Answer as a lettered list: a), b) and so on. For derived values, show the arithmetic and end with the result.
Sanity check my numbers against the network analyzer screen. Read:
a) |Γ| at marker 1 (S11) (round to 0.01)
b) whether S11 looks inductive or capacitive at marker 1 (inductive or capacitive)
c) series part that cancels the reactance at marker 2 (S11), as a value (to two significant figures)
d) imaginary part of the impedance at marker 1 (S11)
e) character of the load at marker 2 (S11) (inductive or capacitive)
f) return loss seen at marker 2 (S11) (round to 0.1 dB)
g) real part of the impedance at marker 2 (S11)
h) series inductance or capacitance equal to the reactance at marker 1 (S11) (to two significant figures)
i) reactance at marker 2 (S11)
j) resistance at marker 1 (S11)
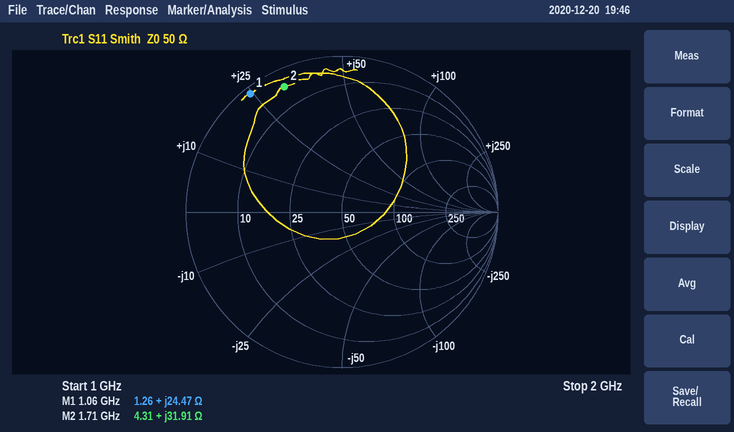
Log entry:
a) 0.96
b) inductive
c) C = 1/(2π × 1.71 GHz × 31.91 Ω) ≈ 2.9 pF
d) +24.47 Ω
e) inductive
f) 1.1 dB
g) 4.31 Ω
h) L = 24.47 Ω/(2π × 1.06 GHz) ≈ 3.7 nH
i) +31.91 Ω
j) 1.26 Ω
